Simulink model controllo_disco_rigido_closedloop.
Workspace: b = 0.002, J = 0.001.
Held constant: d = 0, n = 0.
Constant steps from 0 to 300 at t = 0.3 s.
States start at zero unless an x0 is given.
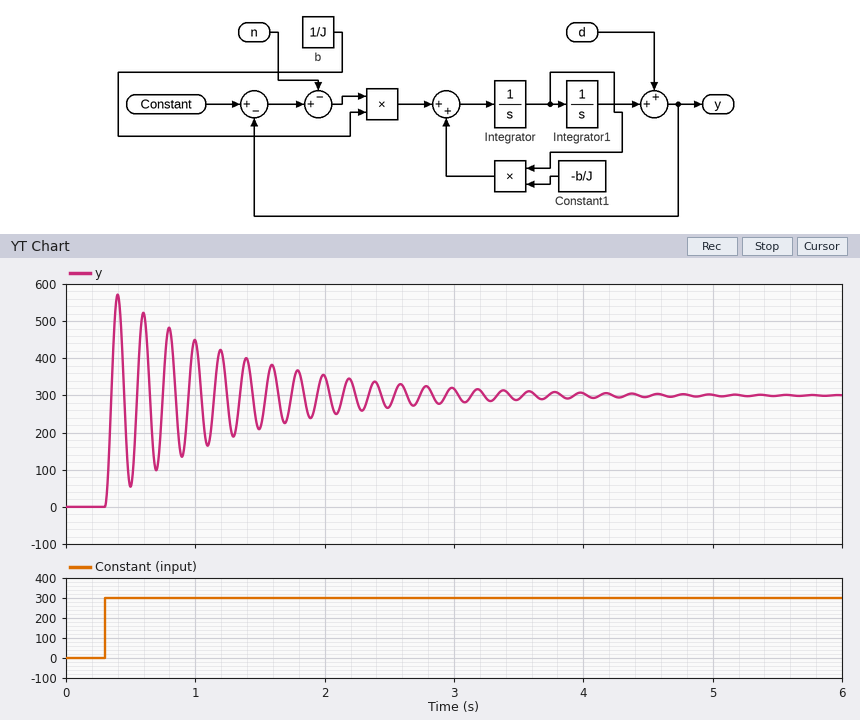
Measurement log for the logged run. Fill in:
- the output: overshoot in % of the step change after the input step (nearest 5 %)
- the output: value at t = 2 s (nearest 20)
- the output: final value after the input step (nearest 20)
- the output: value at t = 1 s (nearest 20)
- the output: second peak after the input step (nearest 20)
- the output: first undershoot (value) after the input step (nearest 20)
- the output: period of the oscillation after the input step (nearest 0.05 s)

90 %
360
300
440
520
60
0.20 s
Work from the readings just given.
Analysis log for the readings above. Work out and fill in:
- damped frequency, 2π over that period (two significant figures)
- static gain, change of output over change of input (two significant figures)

31 rad/s
1.0
